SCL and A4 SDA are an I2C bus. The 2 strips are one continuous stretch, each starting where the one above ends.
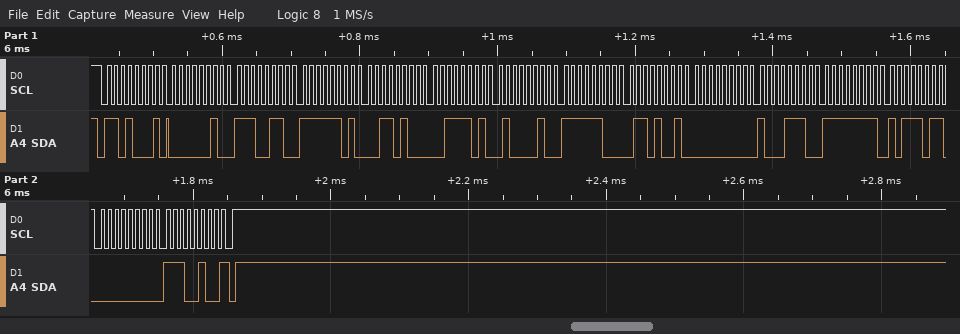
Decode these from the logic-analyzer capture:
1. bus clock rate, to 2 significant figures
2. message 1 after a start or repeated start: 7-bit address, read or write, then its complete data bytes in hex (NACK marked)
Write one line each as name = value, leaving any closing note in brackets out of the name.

bus clock rate, to 2 significant figures = 100 kHz
message 1 after a start or repeated start: 7-bit address, read or write, then its complete data bytes in hex = 0x68 read: 02 E6 FD 34 3D 42 FC 69 00 8E FF BB 00 E4 NACK
